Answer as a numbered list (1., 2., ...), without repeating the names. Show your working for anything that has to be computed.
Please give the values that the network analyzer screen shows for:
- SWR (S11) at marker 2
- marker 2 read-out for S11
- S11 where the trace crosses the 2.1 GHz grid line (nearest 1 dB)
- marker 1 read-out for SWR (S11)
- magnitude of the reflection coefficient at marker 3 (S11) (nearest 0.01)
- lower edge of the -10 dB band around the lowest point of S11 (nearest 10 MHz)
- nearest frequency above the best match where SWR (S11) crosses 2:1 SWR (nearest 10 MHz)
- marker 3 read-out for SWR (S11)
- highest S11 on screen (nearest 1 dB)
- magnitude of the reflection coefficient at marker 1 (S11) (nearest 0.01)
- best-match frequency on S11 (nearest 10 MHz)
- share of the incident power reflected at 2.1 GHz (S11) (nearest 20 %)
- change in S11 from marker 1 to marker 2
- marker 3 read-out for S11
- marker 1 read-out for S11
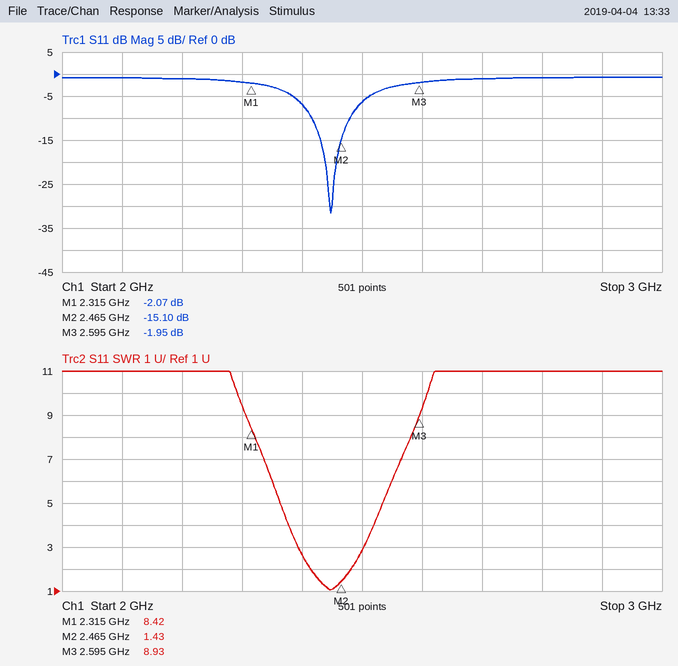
1. 1.43
2. -15.10 dB
3. -1 dB
4. 8.42
5. 10^(-1.95/20) ≈ 0.80
6. 2.42 GHz
7. 2.48 GHz
8. 8.93
9. -1 dB
10. 10^(-2.07/20) ≈ 0.79
11. 2.45 GHz
12. 10^(-1/10) ≈ 79.4 %, so 80 % to the nearest 20 %
13. -15.1 − (-2.07) = -13.03 dB
14. -1.95 dB
15. -2.07 dB
